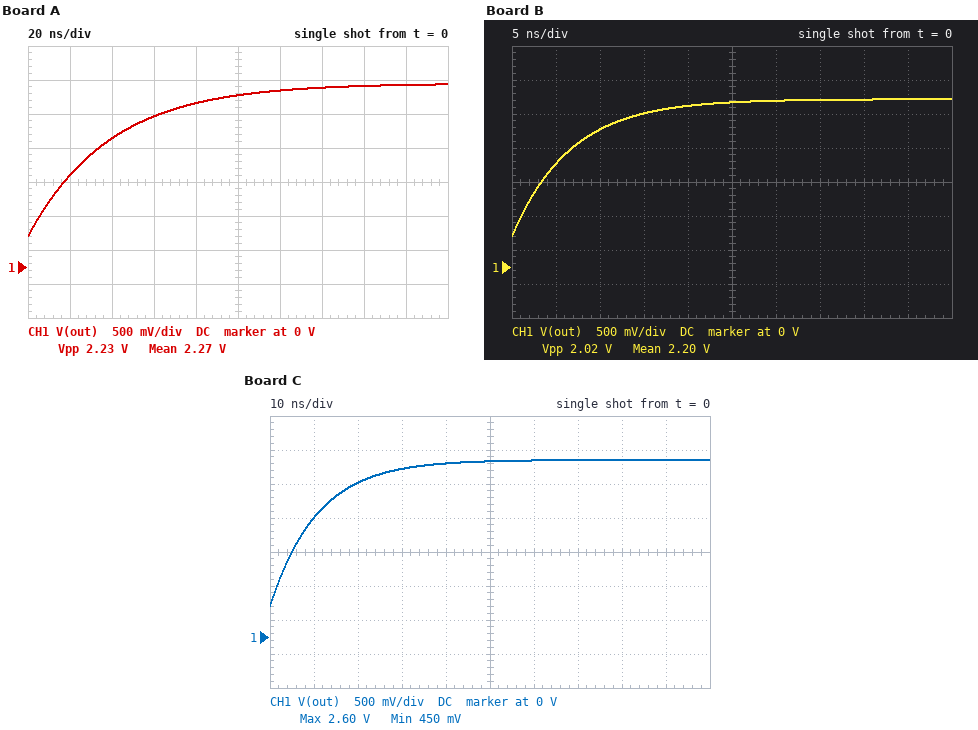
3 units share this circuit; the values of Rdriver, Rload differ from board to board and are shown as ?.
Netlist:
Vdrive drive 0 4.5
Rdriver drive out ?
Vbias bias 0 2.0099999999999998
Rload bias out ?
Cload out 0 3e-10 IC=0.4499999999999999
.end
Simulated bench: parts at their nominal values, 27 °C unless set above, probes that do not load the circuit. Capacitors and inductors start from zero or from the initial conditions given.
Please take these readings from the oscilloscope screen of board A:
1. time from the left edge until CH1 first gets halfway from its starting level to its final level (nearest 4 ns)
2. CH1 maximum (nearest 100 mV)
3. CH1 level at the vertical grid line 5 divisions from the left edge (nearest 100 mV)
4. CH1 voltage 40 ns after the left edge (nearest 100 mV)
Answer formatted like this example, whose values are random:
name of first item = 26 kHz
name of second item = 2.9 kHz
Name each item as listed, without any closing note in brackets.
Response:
time from the left edge until CH1 first gets halfway from its starting level to its final level = 28 ns
CH1 maximum = 2.7 V
CH1 level at the vertical grid line 5 divisions from the left edge = 2.5 V
CH1 voltage 40 ns after the left edge = 1.9 V
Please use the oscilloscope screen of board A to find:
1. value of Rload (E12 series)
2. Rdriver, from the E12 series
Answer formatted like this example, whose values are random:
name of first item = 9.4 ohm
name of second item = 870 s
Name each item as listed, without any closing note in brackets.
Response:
value of Rload = 180 Ω
Rdriver, from the E12 series = 470 Ω
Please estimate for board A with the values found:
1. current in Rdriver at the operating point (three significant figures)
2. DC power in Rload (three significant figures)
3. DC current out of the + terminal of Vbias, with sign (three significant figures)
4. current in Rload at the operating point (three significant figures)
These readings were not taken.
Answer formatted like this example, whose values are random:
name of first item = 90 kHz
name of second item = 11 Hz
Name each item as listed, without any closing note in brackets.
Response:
current in Rdriver at the operating point = 3.83 mA
DC power in Rload = 2.64 mW
DC current out of the + terminal of Vbias, with sign = -3.83 mA
current in Rload at the operating point = 3.83 mA
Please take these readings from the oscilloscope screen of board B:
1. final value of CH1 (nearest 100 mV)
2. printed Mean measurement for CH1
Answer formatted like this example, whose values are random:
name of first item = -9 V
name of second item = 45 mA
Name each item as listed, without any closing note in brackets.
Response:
final value of CH1 = 2.5 V
printed Mean measurement for CH1 = 2.20 V
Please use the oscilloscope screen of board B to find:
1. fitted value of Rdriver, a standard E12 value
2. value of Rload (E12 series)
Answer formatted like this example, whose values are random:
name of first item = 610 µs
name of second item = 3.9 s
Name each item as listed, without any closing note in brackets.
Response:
fitted value of Rdriver, a standard E12 value = 120 Ω
value of Rload = 27 Ω
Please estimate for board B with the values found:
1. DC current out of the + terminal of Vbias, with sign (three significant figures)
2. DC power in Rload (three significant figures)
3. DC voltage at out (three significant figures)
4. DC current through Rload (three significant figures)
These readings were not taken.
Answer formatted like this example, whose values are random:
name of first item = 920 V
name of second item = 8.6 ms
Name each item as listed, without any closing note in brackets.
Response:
DC current out of the + terminal of Vbias, with sign = -16.9 mA
DC power in Rload = 7.75 mW
DC voltage at out = 2.47 V
DC current through Rload = 16.9 mA
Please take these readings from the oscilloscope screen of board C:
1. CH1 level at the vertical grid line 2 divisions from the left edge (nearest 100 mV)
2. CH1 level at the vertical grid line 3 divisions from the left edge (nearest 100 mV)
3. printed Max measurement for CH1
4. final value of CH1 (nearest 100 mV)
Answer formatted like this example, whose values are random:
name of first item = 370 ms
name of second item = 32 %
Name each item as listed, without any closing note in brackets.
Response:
CH1 level at the vertical grid line 2 divisions from the left edge = 2.3 V
CH1 level at the vertical grid line 3 divisions from the left edge = 2.5 V
printed Max measurement for CH1 = 2.60 V
final value of CH1 = 2.6 V
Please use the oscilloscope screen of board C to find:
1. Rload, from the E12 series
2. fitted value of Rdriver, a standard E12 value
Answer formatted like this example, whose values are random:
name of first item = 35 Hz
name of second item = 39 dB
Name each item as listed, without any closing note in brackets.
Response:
Rload, from the E12 series = 47 Ω
fitted value of Rdriver, a standard E12 value = 150 Ω
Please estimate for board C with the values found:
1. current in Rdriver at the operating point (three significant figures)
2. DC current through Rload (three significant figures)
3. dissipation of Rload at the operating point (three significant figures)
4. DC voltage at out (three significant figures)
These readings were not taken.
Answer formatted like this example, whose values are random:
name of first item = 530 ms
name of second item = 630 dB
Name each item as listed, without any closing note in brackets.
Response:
current in Rdriver at the operating point = 12.6 mA
DC current through Rload = 12.6 mA
dissipation of Rload at the operating point = 7.51 mW
DC voltage at out = 2.60 V
